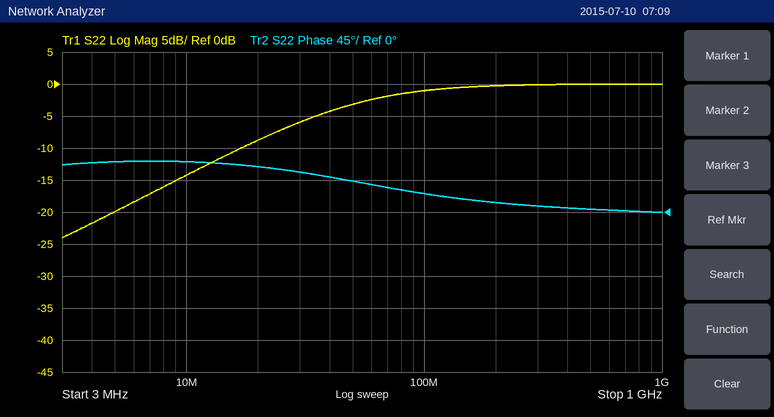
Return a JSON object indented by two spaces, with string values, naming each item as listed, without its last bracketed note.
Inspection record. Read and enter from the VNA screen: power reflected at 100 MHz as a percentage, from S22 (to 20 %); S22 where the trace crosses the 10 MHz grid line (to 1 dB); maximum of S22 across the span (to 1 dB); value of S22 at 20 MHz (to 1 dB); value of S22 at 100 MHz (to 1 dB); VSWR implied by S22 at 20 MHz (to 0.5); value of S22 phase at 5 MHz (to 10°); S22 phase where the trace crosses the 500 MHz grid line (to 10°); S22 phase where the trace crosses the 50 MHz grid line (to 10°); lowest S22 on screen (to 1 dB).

{
  "power reflected at 100 MHz as a percentage, from S22": "80 %",
  "S22 where the trace crosses the 10 MHz grid line": "-14 dB",
  "maximum of S22 across the span": "0 dB",
  "value of S22 at 20 MHz": "-9 dB",
  "value of S22 at 100 MHz": "-1 dB",
  "VSWR implied by S22 at 20 MHz": "2.0",
  "value of S22 phase at 5 MHz": "70°",
  "S22 phase where the trace crosses the 500 MHz grid line": "0°",
  "S22 phase where the trace crosses the 50 MHz grid line": "40°",
  "lowest S22 on screen": "-24 dB"
}
